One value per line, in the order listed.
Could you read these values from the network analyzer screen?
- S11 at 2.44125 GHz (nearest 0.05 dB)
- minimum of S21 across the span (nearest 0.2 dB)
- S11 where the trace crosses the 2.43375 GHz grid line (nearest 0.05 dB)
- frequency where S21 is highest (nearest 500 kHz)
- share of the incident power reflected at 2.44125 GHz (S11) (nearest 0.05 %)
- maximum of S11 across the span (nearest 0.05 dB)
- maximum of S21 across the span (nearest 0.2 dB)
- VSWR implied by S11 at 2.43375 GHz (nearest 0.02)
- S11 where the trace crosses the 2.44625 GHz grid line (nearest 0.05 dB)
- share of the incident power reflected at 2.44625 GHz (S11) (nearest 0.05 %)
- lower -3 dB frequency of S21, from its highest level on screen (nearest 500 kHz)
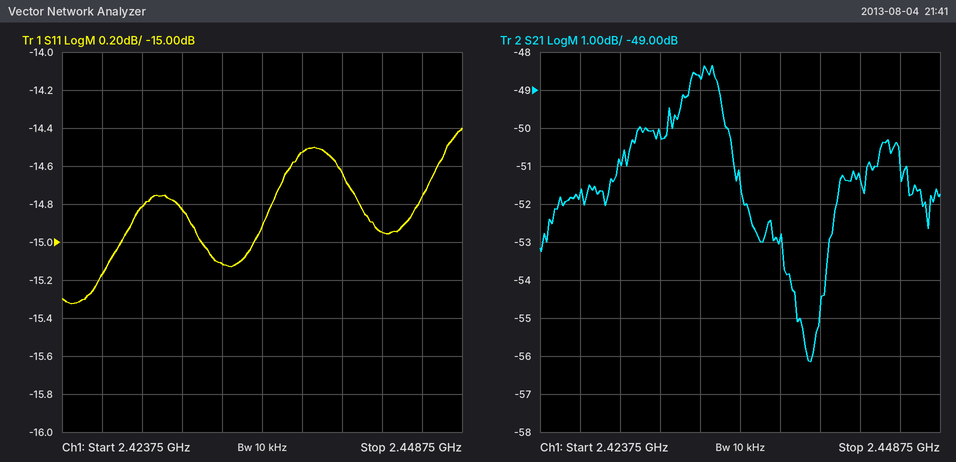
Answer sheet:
-14.65 dB
-56.2 dB
-15.10 dB
2.4345 GHz
3.45 %
-14.40 dB
-48.4 dB
1.42
-14.75 dB
3.35 %
2.4285 GHz
